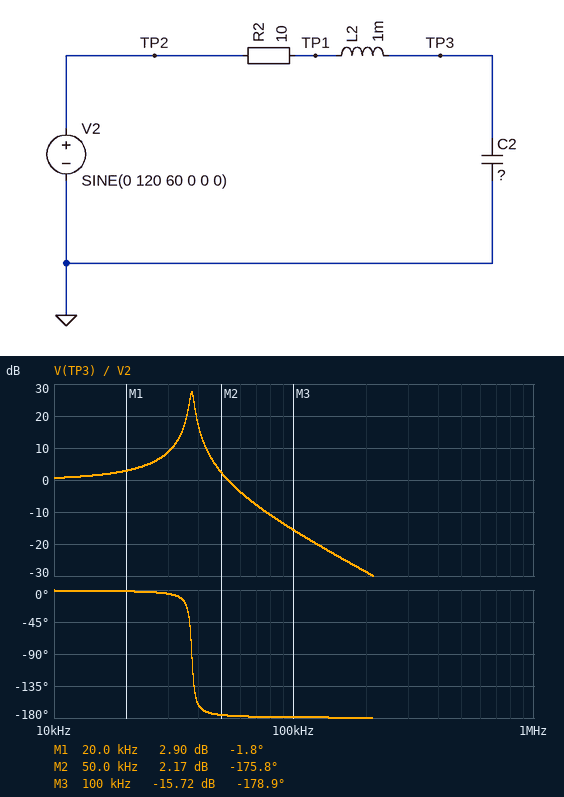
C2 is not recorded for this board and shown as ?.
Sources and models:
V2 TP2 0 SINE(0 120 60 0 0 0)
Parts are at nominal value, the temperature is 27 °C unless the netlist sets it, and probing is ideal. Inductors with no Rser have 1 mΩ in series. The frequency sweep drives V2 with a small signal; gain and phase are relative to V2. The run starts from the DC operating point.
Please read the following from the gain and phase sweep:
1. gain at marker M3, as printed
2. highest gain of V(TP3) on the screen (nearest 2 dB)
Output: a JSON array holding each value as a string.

["-15.72 dB", "28 dB"]
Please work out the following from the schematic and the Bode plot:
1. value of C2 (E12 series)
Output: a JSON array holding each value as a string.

["18 nF"]
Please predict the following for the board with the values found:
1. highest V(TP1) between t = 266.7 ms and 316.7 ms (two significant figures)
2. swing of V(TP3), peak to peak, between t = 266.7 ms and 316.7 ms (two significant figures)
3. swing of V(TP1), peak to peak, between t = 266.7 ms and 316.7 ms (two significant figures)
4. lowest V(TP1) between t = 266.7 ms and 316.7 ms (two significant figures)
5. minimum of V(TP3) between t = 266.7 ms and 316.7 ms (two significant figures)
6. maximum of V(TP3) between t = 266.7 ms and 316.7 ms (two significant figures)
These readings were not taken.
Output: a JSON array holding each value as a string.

["120 V", "240 V", "240 V", "-120 V", "-120 V", "120 V"]
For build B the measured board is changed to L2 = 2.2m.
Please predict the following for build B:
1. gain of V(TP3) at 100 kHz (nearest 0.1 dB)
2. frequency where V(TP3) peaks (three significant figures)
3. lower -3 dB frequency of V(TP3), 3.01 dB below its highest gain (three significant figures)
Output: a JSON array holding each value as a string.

["-23.3 dB", "25.3 kHz", "24.9 kHz"]
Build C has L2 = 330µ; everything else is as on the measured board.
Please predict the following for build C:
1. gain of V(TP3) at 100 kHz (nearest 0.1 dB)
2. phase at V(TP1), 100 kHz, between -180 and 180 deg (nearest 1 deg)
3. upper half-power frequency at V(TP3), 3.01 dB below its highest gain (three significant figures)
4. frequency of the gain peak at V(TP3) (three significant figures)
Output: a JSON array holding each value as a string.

["-2.6 dB", "5 deg", "67.6 kHz", "65.2 kHz"]
